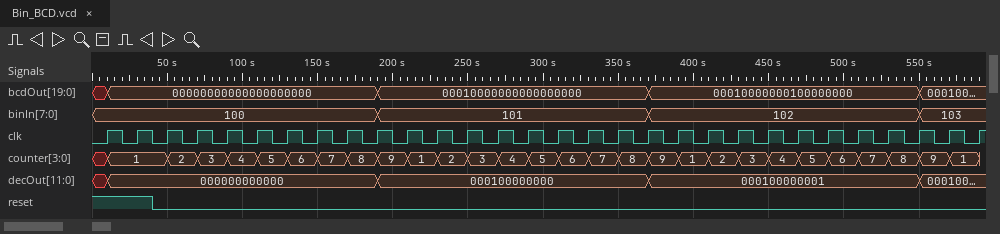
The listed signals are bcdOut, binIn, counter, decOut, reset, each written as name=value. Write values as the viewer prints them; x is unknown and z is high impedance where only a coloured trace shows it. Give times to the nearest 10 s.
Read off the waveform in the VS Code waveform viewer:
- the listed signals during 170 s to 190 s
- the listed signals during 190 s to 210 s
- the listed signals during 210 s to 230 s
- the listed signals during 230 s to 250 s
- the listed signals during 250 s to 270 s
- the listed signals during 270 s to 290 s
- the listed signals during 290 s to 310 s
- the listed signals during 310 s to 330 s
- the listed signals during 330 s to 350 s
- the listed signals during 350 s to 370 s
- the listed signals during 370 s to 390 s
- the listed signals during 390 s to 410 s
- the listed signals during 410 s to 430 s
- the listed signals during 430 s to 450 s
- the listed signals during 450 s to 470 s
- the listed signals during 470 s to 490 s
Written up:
bcdOut=00000000000000000000, binIn=100, counter=8, decOut=000000000000, reset=0
bcdOut=00010000000000000000, binIn=101, counter=9, decOut=000100000000, reset=0
bcdOut=00010000000000000000, binIn=101, counter=1, decOut=000100000000, reset=0
bcdOut=00010000000000000000, binIn=101, counter=2, decOut=000100000000, reset=0
bcdOut=00010000000000000000, binIn=101, counter=3, decOut=000100000000, reset=0
bcdOut=00010000000000000000, binIn=101, counter=4, decOut=000100000000, reset=0
bcdOut=00010000000000000000, binIn=101, counter=5, decOut=000100000000, reset=0
bcdOut=00010000000000000000, binIn=101, counter=6, decOut=000100000000, reset=0
bcdOut=00010000000000000000, binIn=101, counter=7, decOut=000100000000, reset=0
bcdOut=00010000000000000000, binIn=101, counter=8, decOut=000100000000, reset=0
bcdOut=00010000000100000000, binIn=102, counter=9, decOut=000100000001, reset=0
bcdOut=00010000000100000000, binIn=102, counter=1, decOut=000100000001, reset=0
bcdOut=00010000000100000000, binIn=102, counter=2, decOut=000100000001, reset=0
bcdOut=00010000000100000000, binIn=102, counter=3, decOut=000100000001, reset=0
bcdOut=00010000000100000000, binIn=102, counter=4, decOut=000100000001, reset=0
bcdOut=00010000000100000000, binIn=102, counter=5, decOut=000100000001, reset=0
